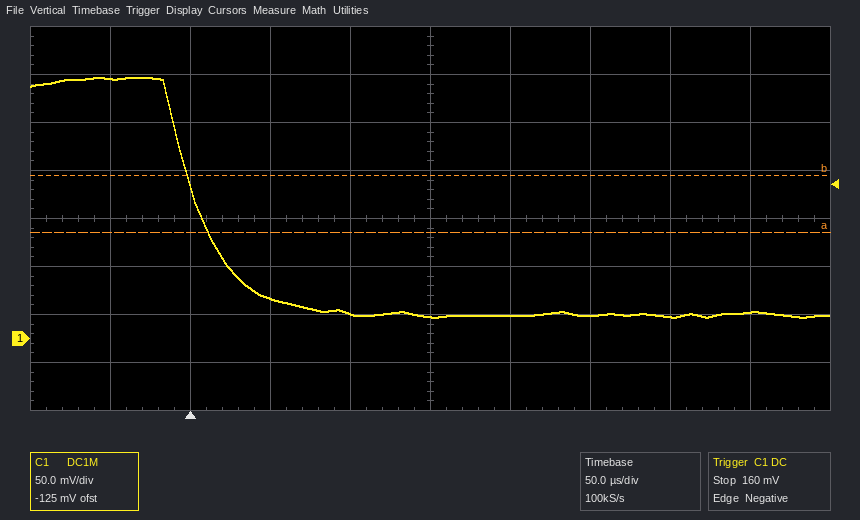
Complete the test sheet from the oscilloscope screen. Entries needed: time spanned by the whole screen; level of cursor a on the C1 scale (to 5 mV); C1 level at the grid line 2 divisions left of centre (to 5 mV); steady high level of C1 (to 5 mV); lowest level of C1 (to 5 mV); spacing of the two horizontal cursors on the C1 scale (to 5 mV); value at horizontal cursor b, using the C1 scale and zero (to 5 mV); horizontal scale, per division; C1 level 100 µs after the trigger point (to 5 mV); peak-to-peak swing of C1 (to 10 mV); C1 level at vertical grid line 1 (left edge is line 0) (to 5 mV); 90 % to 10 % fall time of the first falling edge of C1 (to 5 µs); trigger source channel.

500 µs
110 mV
40 mV
270 mV
20 mV
60 mV
170 mV
50 µs
25 mV
250 mV
270 mV
55 µs
C1
